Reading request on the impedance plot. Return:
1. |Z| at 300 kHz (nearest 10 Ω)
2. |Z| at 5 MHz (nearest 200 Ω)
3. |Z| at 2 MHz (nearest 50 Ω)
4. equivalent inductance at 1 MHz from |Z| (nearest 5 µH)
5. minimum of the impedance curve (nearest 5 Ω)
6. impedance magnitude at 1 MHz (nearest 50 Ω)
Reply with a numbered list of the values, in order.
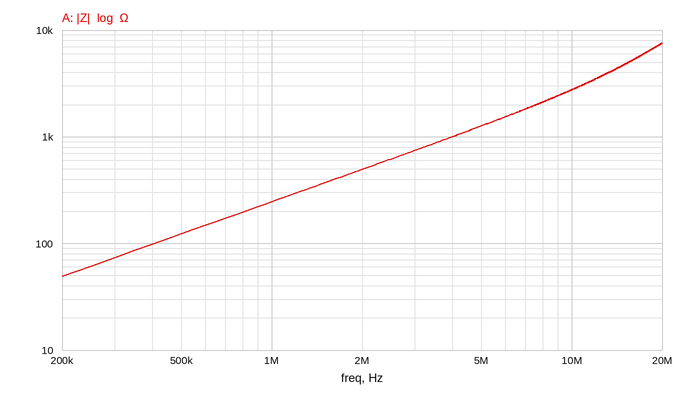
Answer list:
1. 70 Ω
2. 1.2 kΩ
3. 500 Ω
4. 40 µH
5. 50 Ω
6. 250 Ω
